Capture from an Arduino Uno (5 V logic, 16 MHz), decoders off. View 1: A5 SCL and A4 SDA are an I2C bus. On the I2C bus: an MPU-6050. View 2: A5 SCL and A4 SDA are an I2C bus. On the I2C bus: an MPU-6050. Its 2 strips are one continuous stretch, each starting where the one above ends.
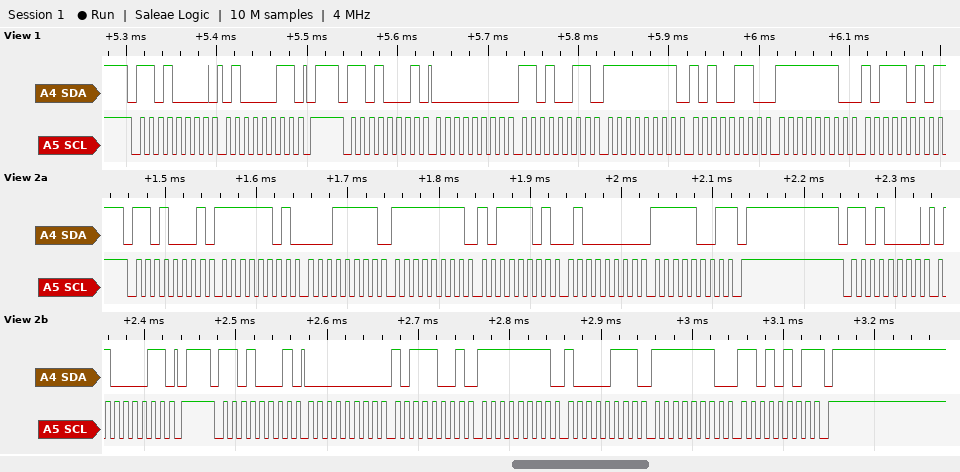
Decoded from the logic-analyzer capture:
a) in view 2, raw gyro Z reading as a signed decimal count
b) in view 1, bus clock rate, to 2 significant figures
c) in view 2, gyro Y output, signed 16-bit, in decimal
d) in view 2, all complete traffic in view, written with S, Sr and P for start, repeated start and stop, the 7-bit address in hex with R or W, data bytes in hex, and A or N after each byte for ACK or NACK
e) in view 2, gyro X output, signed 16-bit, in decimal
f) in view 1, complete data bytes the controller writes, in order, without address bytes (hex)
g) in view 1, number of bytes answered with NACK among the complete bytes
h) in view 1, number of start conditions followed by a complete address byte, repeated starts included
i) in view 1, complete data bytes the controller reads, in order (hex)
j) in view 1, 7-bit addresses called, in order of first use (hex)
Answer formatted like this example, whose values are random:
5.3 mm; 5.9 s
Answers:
-299; 100 kHz; -121; S 68R A FD A 1F A FF A BD A 40 A F9 N P S 68W A 43 A P S 68R A 00 A B9 A FF A 87 A FE A D5 N P; 185; 43; 1; 2; 00 D3 FF A6 FE BA; 0x68
